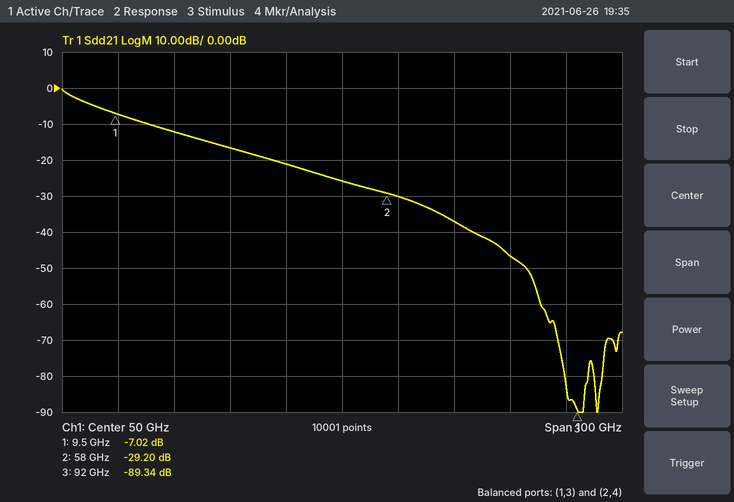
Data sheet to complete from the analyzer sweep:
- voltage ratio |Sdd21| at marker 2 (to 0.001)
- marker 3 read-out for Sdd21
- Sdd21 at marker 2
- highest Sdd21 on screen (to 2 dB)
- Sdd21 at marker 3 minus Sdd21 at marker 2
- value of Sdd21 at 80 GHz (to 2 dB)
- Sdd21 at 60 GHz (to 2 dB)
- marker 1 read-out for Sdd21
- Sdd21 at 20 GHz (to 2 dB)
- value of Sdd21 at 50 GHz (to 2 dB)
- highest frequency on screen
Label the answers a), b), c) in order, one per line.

a) 0.035
b) -89.34 dB
c) -29.20 dB
d) 0 dB
e) -60.14 dB
f) -46 dB
g) -30 dB
h) -7.02 dB
i) -12 dB
j) -26 dB
k) 100 GHz
